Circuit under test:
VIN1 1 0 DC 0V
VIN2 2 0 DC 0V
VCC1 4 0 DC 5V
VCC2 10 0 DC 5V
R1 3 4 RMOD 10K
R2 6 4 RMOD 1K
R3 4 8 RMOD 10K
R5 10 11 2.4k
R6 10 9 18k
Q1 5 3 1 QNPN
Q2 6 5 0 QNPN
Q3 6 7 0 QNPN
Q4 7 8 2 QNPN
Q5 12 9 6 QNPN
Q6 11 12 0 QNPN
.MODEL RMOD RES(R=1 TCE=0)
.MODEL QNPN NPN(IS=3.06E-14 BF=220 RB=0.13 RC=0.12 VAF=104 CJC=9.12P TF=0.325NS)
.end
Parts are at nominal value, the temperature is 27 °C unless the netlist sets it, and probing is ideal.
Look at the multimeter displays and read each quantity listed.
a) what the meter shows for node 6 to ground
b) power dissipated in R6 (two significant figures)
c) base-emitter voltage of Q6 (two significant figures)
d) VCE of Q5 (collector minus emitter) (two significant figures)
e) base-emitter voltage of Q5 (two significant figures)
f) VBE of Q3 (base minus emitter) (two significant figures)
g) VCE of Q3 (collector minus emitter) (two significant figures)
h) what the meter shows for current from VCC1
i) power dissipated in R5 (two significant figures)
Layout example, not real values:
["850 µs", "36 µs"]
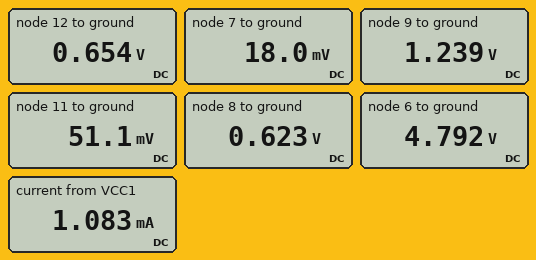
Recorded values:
["4.792 V", "790 µW", "650 mV", "-4.1 V", "-3.6 V", "18 mV", "4.8 V", "1.083 mA", "10 mW"]
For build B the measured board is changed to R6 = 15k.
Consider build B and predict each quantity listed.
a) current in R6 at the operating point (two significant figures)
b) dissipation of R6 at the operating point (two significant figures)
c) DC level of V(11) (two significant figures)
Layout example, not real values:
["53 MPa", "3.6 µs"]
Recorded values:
["250 µA", "940 µW", "48 mV"]
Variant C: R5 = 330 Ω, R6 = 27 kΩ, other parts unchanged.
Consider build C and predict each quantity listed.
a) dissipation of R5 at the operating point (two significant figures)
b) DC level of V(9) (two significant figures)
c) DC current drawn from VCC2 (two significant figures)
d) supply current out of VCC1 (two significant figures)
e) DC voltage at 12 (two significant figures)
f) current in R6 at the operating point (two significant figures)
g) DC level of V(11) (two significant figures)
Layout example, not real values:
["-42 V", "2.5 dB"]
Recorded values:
["72 mW", "1.3 V", "15 mA", "1.0 mA", "700 mV", "140 µA", "110 mV"]
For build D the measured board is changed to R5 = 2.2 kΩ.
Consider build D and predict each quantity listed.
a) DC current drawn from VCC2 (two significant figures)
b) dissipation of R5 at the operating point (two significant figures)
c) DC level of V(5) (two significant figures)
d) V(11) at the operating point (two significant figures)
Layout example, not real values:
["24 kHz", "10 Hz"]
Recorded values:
["2.5 mA", "11 mW", "18 mV", "53 mV"]
